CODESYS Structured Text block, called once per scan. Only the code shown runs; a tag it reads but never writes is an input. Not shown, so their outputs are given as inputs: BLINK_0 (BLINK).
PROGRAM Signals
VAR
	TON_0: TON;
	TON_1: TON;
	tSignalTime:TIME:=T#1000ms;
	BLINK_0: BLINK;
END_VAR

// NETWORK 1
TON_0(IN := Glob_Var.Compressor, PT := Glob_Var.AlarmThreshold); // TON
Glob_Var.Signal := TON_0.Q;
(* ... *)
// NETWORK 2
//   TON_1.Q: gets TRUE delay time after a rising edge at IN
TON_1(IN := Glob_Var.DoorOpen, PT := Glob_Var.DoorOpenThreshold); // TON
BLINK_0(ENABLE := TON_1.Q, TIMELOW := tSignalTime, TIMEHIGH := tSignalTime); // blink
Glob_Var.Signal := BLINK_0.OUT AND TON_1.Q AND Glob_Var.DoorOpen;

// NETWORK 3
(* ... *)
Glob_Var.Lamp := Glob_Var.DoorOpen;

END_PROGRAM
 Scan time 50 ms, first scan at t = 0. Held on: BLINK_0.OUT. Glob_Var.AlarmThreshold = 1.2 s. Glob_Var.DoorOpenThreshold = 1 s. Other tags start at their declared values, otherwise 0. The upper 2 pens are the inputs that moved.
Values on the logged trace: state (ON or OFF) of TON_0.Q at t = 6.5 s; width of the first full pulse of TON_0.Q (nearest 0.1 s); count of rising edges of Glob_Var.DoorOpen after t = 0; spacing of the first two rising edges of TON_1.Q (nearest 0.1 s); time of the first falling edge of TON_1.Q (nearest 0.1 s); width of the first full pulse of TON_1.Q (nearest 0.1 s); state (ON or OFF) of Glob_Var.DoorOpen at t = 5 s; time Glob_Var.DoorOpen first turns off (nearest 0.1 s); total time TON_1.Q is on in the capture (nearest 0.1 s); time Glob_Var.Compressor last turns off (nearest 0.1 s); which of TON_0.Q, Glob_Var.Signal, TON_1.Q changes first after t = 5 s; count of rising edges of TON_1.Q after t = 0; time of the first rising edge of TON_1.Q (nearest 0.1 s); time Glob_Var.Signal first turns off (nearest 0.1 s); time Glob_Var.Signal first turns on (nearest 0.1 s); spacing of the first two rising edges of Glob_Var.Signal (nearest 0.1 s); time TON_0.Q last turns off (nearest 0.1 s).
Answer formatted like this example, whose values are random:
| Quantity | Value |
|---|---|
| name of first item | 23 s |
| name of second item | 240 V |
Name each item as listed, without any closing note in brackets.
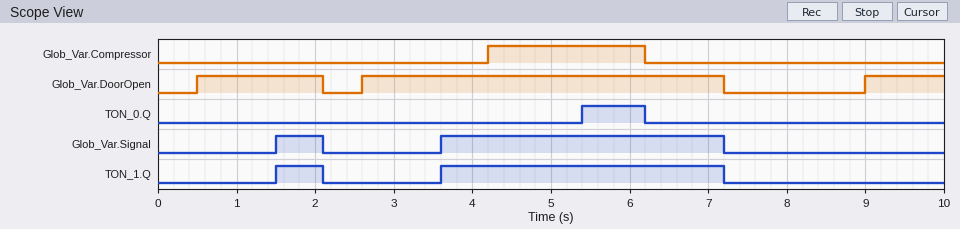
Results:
| Quantity | Value |
|---|---|
| state (ON or OFF) of TON_0.Q at t = 6.5 s | OFF |
| width of the first full pulse of TON_0.Q | 0.8 s |
| count of rising edges of Glob_Var.DoorOpen after t = 0 | 3 |
| spacing of the first two rising edges of TON_1.Q | 2.1 s |
| time of the first falling edge of TON_1.Q | 2.1 s |
| width of the first full pulse of TON_1.Q | 0.6 s |
| state (ON or OFF) of Glob_Var.DoorOpen at t = 5 s | ON |
| time Glob_Var.DoorOpen first turns off | 2.1 s |
| total time TON_1.Q is on in the capture | 4.2 s |
| time Glob_Var.Compressor last turns off | 6.2 s |
| which of TON_0.Q, Glob_Var.Signal, TON_1.Q changes first after t = 5 s | TON_0.Q |
| count of rising edges of TON_1.Q after t = 0 | 2 |
| time of the first rising edge of TON_1.Q | 1.5 s |
| time Glob_Var.Signal first turns off | 2.1 s |
| time Glob_Var.Signal first turns on | 1.5 s |
| spacing of the first two rising edges of Glob_Var.Signal | 2.1 s |
| time TON_0.Q last turns off | 6.2 s |
